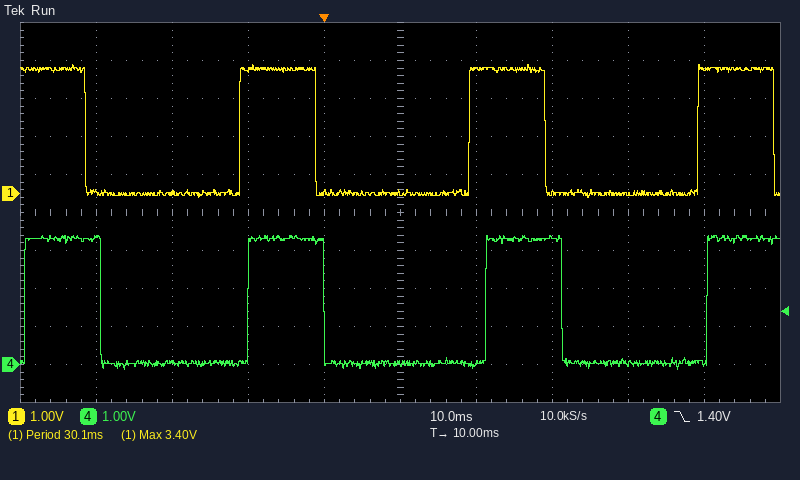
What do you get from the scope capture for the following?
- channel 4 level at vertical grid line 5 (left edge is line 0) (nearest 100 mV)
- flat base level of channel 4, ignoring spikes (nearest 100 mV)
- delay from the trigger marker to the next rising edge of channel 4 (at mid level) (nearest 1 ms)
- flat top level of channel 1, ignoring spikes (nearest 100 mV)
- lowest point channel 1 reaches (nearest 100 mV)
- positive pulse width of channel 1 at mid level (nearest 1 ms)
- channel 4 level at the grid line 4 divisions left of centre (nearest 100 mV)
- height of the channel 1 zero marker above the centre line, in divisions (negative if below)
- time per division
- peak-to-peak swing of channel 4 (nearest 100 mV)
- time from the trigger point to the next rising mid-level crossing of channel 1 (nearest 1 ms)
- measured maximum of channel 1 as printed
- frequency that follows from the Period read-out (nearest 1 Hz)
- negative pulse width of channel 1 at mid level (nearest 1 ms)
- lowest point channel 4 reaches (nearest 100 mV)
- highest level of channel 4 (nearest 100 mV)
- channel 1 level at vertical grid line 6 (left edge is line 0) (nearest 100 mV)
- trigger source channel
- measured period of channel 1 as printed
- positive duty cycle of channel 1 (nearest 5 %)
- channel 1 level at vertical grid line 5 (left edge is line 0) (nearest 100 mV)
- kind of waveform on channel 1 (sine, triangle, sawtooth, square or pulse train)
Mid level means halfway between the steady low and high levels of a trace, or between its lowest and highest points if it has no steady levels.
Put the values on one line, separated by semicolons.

0.0 V; 0.0 V; 21 ms; 3.3 V; -100 mV; 10 ms; 3.3 V; +0.5 div; 10 ms; 3.5 V; 19 ms; 3.40 V; 33 Hz; 20 ms; -100 mV; 3.4 V; 3.3 V; channel 4; 30.1 ms; 35 %; 0.0 V; pulse train
